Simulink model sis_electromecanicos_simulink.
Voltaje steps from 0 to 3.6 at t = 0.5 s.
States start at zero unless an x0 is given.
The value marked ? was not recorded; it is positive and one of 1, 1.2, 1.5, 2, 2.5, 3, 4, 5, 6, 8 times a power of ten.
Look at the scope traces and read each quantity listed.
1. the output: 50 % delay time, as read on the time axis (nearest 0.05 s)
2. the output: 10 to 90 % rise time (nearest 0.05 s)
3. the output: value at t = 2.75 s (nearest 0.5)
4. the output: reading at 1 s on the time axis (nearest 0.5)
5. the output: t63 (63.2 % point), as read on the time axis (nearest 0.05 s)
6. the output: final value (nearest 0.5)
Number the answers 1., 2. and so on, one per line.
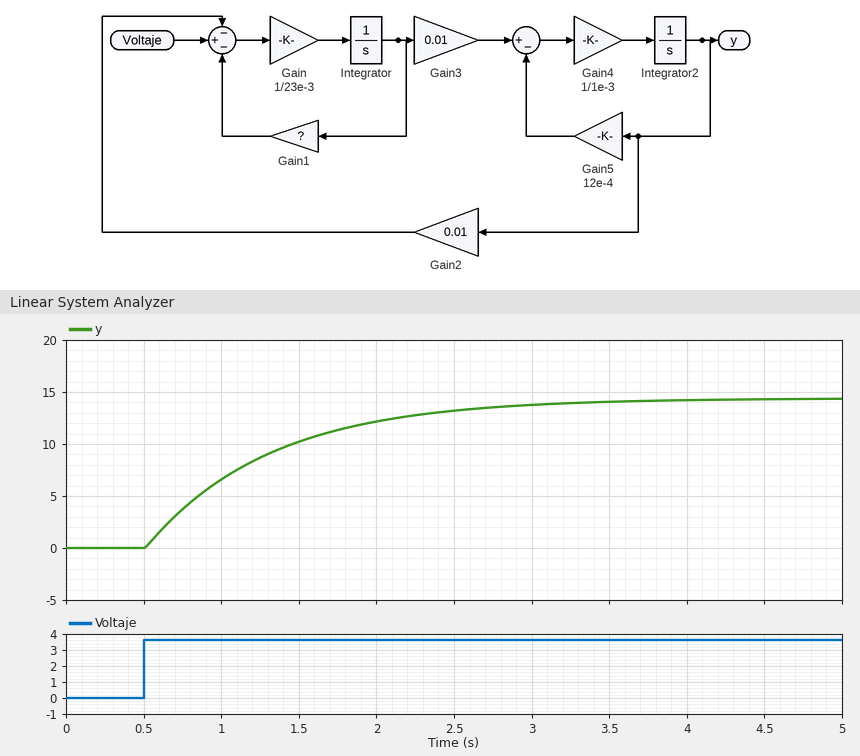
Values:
1. 1.05 s
2. 1.75 s
3. 13.5
4. 6.5
5. 1.30 s
6. 14.5
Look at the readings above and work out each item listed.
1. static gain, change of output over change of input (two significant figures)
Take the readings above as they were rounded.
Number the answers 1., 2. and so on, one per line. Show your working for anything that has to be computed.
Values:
1. (14.5 - 0) / (3.6 - 0) = 4.0
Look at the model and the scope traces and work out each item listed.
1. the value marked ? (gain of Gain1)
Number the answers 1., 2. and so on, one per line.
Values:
1. 2
